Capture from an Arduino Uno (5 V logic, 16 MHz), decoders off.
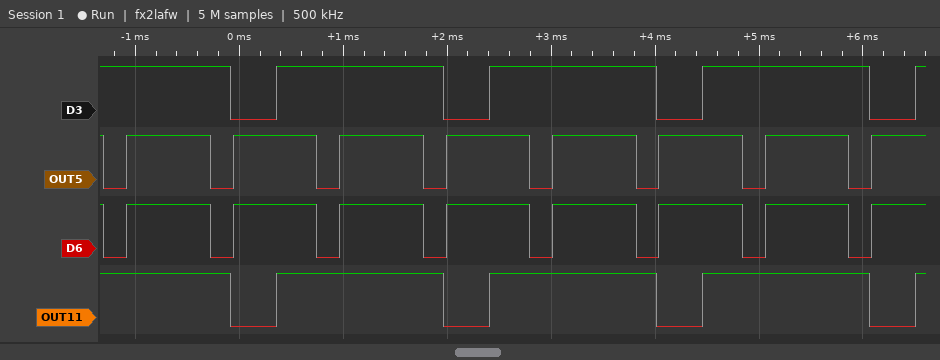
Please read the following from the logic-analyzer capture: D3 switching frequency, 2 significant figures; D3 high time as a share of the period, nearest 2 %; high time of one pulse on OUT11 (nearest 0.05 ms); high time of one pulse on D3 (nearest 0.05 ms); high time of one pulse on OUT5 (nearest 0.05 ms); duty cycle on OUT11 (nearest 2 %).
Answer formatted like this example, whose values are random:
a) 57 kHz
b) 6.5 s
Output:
a) 490 Hz
b) 78 %
c) 1.60 ms
d) 1.60 ms
e) 0.80 ms
f) 78 %
